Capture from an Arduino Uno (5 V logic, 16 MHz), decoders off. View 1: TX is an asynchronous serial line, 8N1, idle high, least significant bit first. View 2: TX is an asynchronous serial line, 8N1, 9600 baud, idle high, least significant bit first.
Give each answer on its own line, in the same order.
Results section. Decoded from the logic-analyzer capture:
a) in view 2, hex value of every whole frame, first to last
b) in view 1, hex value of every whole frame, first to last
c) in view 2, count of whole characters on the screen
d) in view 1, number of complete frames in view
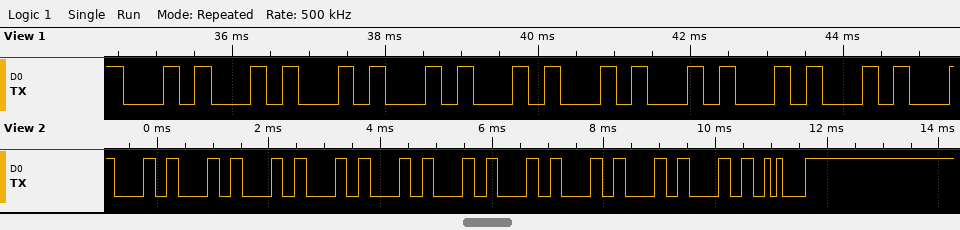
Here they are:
0x30 0x30 0x30 0x30 0x30 0x30 0x30 0x30 0x30 0x30 0x0A
0x30 0x30 0x30 0x30 0x30 0x30 0x30 0x30 0x30
11
9
